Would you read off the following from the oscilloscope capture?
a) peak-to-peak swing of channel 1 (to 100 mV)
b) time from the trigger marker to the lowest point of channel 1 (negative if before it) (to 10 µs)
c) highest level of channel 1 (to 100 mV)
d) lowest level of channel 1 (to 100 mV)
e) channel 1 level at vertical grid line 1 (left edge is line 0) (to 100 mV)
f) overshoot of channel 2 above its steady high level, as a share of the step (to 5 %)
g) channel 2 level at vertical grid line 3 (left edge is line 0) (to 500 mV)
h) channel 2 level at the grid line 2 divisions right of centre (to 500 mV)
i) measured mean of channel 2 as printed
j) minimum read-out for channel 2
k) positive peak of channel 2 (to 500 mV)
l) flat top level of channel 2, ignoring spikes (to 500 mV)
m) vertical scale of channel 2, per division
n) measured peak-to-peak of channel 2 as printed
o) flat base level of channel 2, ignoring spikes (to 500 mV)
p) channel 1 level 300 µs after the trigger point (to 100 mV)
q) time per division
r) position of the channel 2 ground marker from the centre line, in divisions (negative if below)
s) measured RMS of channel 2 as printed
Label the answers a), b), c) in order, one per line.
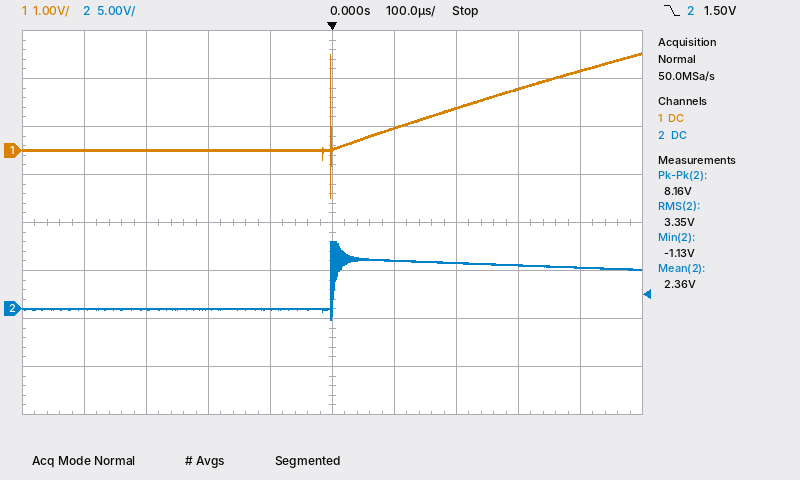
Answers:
a) 3.0 V
b) 0 µs
c) 2.0 V
d) -1.0 V
e) 0.0 V
f) 55 %
g) 0.0 V
h) 5.0 V
i) 2.36 V
j) -1.13 V
k) 7.0 V
l) 4.5 V
m) 5 V
n) 8.16 V
o) 0.0 V
p) 1.3 V
q) 100 µs
r) -1.8 div
s) 3.35 V
